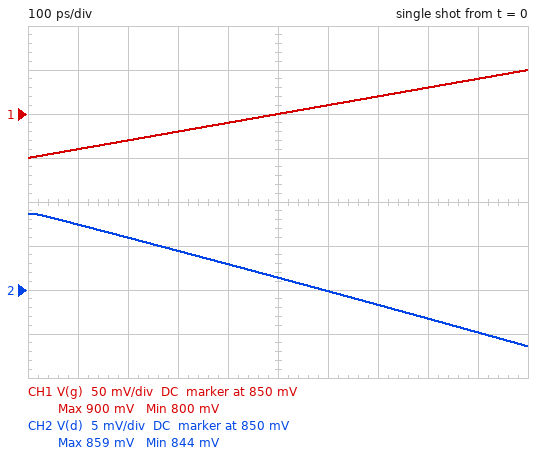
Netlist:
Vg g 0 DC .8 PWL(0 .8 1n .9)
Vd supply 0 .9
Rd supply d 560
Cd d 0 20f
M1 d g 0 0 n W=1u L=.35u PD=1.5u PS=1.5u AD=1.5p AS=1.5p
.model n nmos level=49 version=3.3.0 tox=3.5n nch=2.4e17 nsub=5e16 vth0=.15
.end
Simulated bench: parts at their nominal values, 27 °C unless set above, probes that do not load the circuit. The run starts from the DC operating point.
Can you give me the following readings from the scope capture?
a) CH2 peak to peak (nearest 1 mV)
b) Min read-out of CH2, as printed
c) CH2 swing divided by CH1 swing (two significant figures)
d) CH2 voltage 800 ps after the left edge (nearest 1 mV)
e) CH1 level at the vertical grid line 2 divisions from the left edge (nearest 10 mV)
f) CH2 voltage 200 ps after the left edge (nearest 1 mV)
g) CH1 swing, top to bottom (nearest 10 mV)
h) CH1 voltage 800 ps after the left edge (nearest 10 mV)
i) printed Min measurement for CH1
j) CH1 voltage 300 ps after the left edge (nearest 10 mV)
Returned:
15 mV
844 mV
0.15
847 mV
820 mV
856 mV
100 mV
880 mV
800 mV
830 mV
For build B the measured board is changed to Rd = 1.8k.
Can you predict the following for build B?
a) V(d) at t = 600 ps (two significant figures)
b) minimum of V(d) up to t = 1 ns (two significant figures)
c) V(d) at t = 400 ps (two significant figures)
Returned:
740 mV
720 mV
750 mV
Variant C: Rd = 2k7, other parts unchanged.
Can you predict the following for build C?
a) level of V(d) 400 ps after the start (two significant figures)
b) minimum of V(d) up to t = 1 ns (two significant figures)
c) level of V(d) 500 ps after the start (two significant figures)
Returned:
680 mV
640 mV
670 mV
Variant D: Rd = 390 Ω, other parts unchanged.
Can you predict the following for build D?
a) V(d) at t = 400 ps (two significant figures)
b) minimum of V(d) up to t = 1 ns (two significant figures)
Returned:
870 mV
860 mV
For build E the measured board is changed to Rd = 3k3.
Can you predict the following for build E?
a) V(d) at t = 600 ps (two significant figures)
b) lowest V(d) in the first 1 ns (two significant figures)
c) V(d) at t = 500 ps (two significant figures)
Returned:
620 mV
580 mV
630 mV
